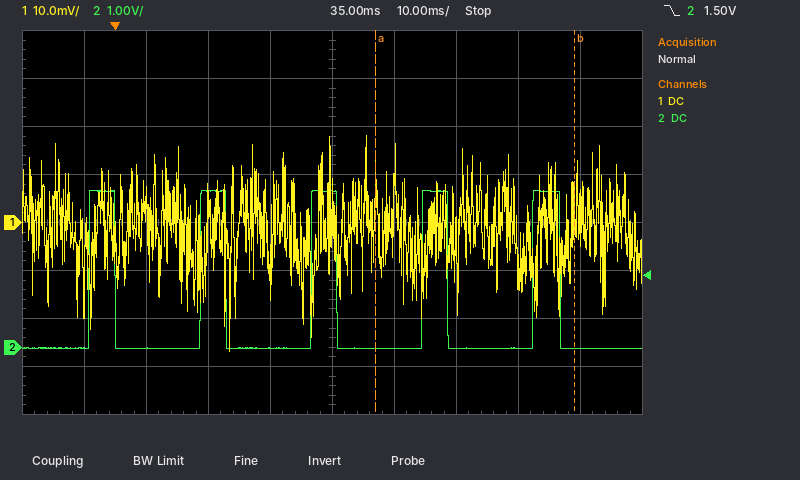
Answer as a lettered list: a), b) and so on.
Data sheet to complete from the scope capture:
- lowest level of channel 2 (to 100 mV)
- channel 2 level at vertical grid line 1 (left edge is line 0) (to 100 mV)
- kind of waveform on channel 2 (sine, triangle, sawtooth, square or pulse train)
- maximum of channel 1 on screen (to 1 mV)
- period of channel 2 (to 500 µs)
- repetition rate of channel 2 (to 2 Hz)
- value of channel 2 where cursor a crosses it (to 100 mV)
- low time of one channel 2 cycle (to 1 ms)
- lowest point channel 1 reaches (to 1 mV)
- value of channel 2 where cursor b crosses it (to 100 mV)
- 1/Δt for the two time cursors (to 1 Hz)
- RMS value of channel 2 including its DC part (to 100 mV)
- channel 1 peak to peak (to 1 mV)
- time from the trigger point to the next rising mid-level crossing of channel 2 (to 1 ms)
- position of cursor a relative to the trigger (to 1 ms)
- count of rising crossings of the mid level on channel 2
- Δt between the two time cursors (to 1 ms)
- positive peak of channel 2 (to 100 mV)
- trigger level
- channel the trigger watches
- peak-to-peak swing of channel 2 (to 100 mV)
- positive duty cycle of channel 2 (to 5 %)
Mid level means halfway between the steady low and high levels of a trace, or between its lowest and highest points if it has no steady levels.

a) 0.0 V
b) 0.0 V
c) pulse train
d) 18 mV
e) 18.0 ms
f) 56 Hz
g) 0.0 V
h) 14 ms
i) -27 mV
j) 0.0 V
k) 31 Hz
l) 1.6 V
m) 45 mV
n) 14 ms
o) +42 ms
p) 5
q) 32 ms
r) 3.3 V
s) 1.50 V
t) channel 2
u) 3.3 V
v) 25 %
